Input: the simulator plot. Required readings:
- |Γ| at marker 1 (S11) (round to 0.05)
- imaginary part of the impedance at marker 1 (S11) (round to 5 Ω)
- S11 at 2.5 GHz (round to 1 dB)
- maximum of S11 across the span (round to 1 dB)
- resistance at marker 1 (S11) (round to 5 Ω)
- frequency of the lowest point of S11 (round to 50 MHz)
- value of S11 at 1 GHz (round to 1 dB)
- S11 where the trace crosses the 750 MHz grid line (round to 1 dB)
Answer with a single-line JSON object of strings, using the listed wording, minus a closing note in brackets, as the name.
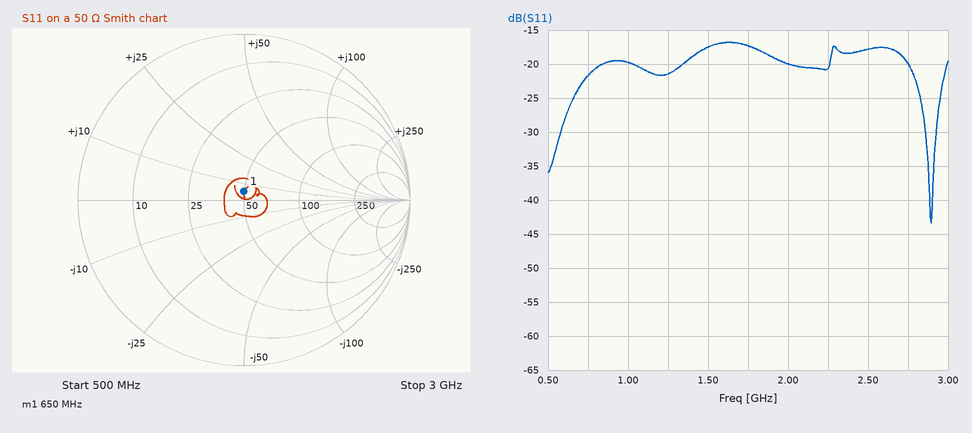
{"|Γ| at marker 1 (S11)": "0.05", "imaginary part of the impedance at marker 1 (S11)": "+5 Ω", "S11 at 2.5 GHz": "-18 dB", "maximum of S11 across the span": "-17 dB", "resistance at marker 1 (S11)": "50 Ω", "frequency of the lowest point of S11": "2.90 GHz", "value of S11 at 1 GHz": "-20 dB", "S11 where the trace crosses the 750 MHz grid line": "-22 dB"}
